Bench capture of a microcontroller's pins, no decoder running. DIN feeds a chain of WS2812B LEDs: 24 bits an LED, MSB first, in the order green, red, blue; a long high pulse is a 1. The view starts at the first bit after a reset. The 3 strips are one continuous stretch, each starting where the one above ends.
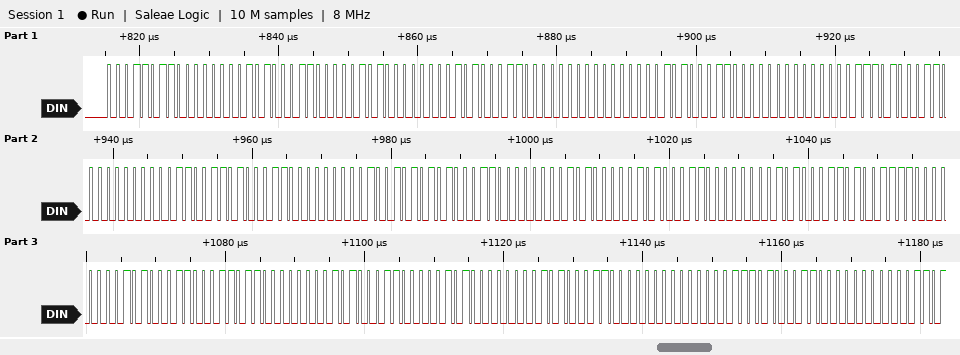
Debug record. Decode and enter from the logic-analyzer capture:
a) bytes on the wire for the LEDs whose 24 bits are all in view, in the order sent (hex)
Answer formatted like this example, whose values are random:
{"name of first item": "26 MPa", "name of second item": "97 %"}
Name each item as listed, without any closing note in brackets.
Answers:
{"bytes on the wire for the LEDs whose 24 bits are all in view, in the order sent": "1B 00 A3 05 00 A3 00 00 A3 00 03 A3 00 19 A3 00 4A A3 00 A0 A3 00 A3 4F 00 A3 1B 00 A3 05 00 A3 00 03 A3 00"}
